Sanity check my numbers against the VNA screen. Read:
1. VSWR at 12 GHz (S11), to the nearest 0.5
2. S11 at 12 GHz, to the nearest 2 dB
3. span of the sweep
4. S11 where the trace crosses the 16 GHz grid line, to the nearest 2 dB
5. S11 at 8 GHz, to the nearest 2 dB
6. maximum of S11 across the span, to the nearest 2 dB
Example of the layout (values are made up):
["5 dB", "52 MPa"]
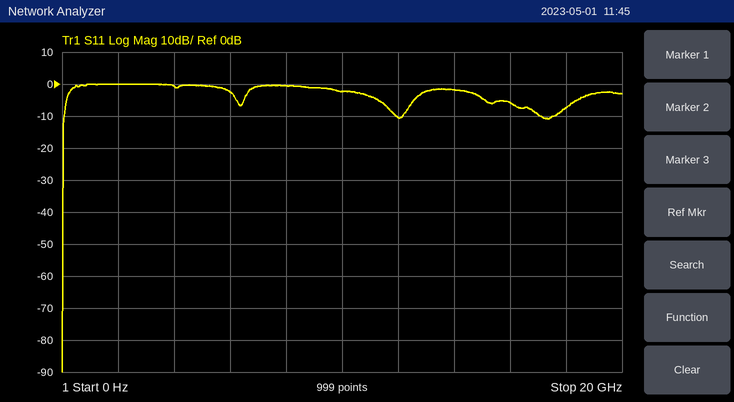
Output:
["2.0", "-10 dB", "20 GHz", "-6 dB", "0 dB", "0 dB"]
